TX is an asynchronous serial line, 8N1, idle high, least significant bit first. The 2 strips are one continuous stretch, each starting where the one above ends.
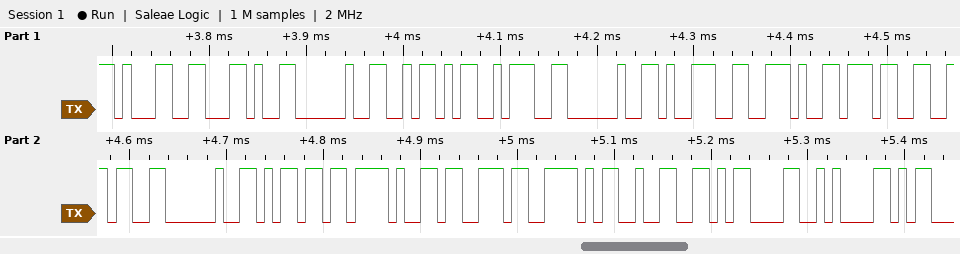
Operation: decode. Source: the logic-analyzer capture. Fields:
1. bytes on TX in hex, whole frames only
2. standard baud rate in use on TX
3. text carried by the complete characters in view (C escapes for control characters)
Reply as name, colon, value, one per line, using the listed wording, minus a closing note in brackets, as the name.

bytes on TX in hex, whole frames only: 0x31 0x2C 0x20 0x5A 0x3A 0x20 0x39 0x2E 0x37 0x36 0x20 0x6D 0x2F 0x73 0x5E 0x32 0x0D 0x0A
standard baud rate in use on TX: 115200 baud
text carried by the complete characters in view: "1, Z: 9.76 m/s^2\r\n"
